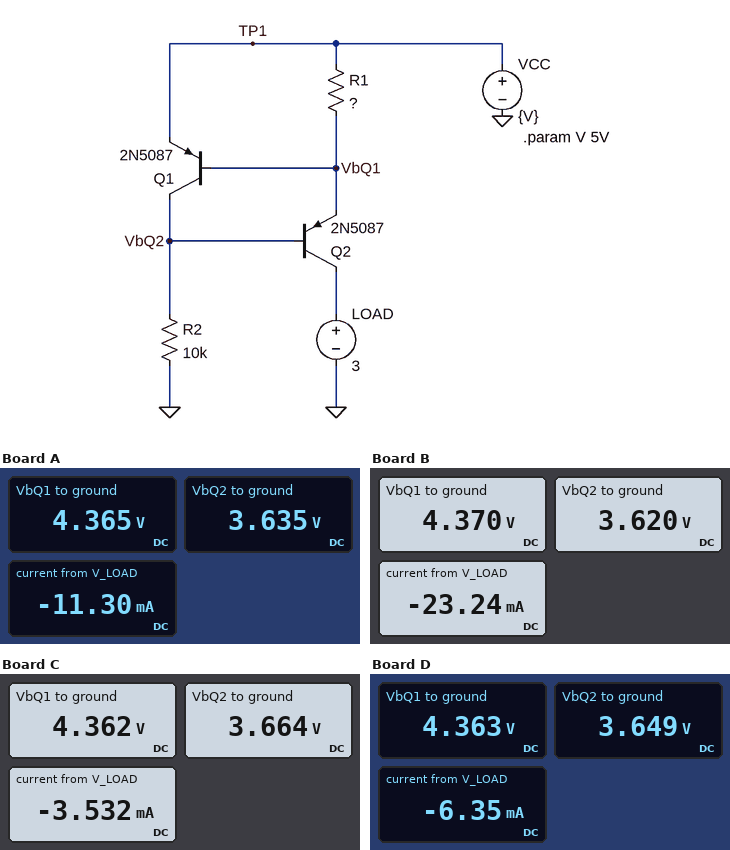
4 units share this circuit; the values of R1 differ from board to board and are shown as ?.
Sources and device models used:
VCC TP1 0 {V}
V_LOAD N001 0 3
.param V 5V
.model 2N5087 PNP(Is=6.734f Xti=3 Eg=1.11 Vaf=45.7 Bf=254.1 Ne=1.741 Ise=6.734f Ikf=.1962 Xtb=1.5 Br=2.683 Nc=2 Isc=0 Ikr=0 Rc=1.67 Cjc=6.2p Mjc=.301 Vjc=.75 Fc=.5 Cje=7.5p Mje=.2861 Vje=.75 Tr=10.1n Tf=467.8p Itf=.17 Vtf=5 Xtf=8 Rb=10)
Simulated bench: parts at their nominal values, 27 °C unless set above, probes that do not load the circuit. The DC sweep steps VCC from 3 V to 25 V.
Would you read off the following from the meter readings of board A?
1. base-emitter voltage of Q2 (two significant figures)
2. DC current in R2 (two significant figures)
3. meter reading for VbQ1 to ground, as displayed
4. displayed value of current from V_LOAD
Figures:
-730 mV
360 µA
4.365 V
-11.30 mA
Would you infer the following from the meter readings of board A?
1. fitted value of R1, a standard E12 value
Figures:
56 Ω
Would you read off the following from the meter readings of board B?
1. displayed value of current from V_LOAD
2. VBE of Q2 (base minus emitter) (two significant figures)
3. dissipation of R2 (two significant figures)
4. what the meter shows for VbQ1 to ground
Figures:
-23.24 mA
-750 mV
1.3 mW
4.370 V
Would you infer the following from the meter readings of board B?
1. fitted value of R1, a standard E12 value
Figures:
27 Ω
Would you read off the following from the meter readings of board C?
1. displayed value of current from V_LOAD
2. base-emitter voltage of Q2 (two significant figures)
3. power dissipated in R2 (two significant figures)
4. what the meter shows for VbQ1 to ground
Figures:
-3.532 mA
-700 mV
1.3 mW
4.362 V
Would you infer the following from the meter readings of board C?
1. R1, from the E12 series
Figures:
180 Ω
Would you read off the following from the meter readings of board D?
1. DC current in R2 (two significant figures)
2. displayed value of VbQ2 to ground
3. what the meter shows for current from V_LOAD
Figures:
360 µA
3.649 V
-6.35 mA
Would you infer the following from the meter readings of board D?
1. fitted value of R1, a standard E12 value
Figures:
100 Ω
